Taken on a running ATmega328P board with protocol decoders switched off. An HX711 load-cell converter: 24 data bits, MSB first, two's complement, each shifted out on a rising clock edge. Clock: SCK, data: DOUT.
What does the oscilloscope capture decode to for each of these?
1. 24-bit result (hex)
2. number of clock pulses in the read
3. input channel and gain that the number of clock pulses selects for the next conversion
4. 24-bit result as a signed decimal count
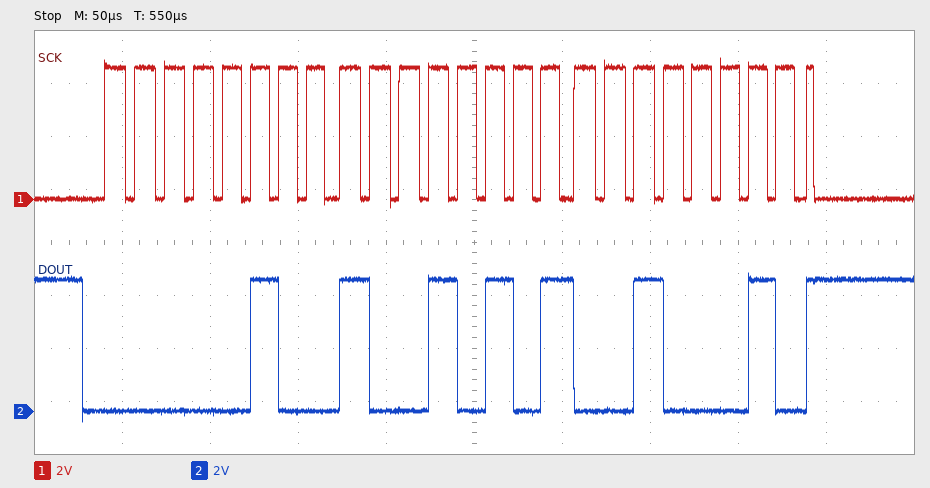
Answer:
0x049522
25
channel A, gain 128
300322
